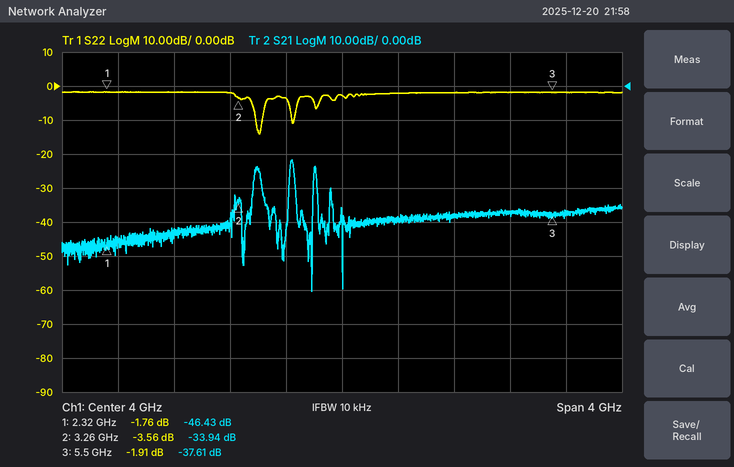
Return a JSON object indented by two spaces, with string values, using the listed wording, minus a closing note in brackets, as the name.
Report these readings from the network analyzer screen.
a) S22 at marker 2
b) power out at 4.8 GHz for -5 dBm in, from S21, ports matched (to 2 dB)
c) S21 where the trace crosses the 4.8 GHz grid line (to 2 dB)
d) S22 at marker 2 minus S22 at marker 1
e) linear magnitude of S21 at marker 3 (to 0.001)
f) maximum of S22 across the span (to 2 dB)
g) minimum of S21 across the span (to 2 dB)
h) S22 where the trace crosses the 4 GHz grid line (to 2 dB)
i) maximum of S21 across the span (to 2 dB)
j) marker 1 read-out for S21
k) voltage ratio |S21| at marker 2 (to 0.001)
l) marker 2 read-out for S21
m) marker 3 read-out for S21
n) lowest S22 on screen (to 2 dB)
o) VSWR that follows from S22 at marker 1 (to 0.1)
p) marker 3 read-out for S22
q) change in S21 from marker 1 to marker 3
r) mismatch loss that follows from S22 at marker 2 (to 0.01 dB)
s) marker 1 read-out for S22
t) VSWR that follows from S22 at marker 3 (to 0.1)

{
  "S22 at marker 2": "-3.56 dB",
  "power out at 4.8 GHz for -5 dBm in, from S21, ports matched": "-44 dBm",
  "S21 where the trace crosses the 4.8 GHz grid line": "-38 dB",
  "S22 at marker 2 minus S22 at marker 1": "-1.80 dB",
  "linear magnitude of S21 at marker 3": "0.013",
  "maximum of S22 across the span": "-2 dB",
  "minimum of S21 across the span": "-60 dB",
  "S22 where the trace crosses the 4 GHz grid line": "-2 dB",
  "maximum of S21 across the span": "-22 dB",
  "marker 1 read-out for S21": "-46.43 dB",
  "voltage ratio |S21| at marker 2": "0.020",
  "marker 2 read-out for S21": "-33.94 dB",
  "marker 3 read-out for S21": "-37.61 dB",
  "lowest S22 on screen": "-14 dB",
  "VSWR that follows from S22 at marker 1": "9.9",
  "marker 3 read-out for S22": "-1.91 dB",
  "change in S21 from marker 1 to marker 3": "8.82 dB",
  "mismatch loss that follows from S22 at marker 2": "2.52 dB",
  "marker 1 read-out for S22": "-1.76 dB",
  "VSWR that follows from S22 at marker 3": "9.1"
}
